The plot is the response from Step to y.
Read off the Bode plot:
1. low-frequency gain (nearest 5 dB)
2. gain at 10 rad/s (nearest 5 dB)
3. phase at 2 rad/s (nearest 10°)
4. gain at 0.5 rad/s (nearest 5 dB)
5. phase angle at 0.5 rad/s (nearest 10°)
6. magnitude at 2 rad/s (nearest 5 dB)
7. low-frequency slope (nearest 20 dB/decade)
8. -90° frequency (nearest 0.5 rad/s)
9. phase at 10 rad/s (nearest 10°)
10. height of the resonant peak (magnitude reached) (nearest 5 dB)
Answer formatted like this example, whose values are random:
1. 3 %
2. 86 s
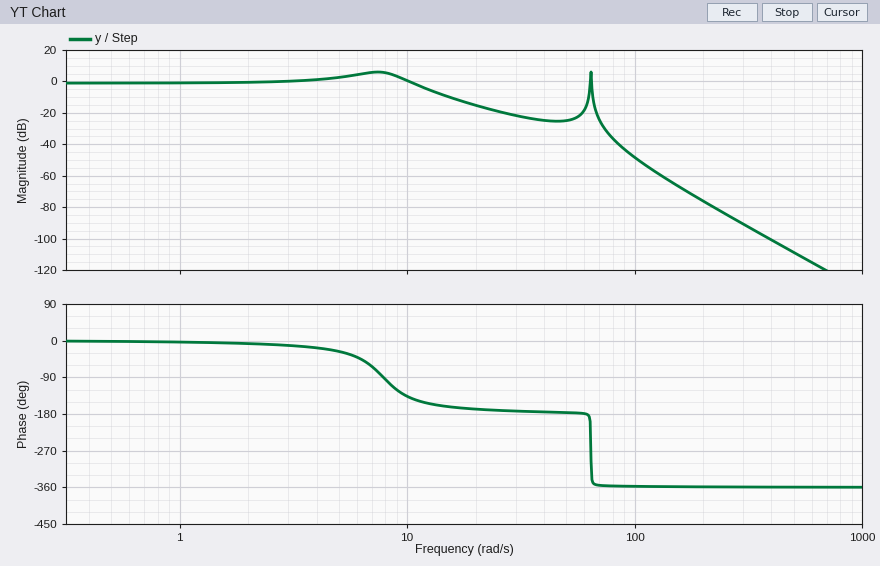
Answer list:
1. 0 dB
2. 0 dB
3. -10°
4. 0 dB
5. 0°
6. 0 dB
7. 0 dB/decade
8. 8.0 rad/s
9. -140°
10. 5 dB
